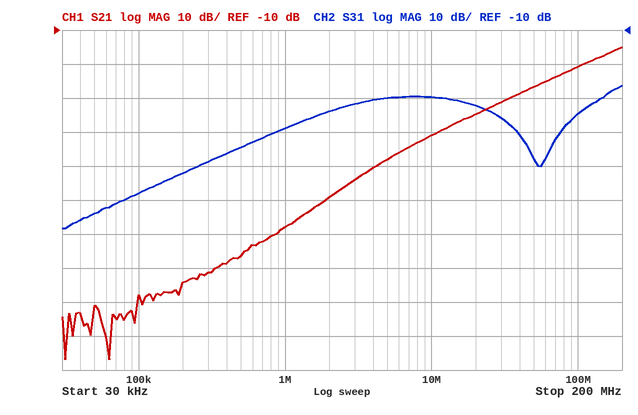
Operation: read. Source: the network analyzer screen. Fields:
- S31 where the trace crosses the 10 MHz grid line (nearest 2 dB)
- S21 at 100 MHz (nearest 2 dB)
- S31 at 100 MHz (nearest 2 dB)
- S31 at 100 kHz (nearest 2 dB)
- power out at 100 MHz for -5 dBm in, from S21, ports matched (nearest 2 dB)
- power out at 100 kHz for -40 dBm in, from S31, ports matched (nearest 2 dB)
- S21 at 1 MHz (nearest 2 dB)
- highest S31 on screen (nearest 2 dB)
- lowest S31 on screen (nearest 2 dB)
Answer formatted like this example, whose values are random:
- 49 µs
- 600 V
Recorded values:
- -30 dB
- -20 dB
- -34 dB
- -58 dB
- -26 dBm
- -98 dBm
- -68 dB
- -26 dB
- -68 dB
